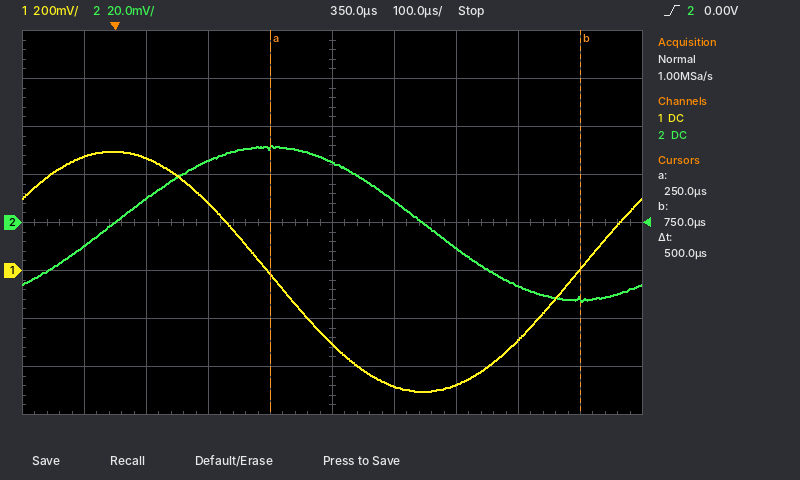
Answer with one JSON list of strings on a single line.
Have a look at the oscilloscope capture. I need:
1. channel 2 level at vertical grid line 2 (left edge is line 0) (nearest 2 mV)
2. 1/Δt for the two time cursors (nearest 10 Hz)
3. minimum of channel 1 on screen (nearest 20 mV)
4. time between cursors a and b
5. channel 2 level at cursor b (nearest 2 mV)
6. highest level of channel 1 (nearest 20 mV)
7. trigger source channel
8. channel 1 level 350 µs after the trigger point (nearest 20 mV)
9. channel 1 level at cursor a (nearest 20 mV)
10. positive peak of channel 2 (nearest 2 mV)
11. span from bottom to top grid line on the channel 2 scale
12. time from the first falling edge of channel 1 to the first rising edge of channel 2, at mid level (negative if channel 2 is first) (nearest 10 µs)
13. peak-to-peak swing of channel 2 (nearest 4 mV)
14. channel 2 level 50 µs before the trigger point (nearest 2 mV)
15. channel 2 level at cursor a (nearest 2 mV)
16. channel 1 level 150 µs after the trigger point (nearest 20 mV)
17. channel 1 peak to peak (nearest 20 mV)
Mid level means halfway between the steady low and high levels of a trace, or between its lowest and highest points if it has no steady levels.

["10 mV", "2.00 kHz", "-500 mV", "500 µs", "-32 mV", "500 mV", "channel 2", "-300 mV", "-20 mV", "32 mV", "160 mV", "-250 µs", "64 mV", "-10 mV", "32 mV", "280 mV", "1.00 V"]
